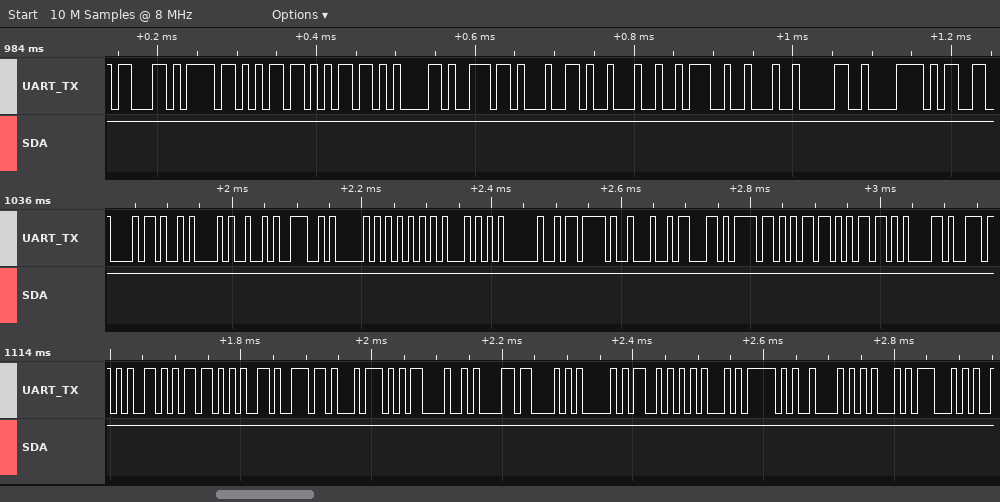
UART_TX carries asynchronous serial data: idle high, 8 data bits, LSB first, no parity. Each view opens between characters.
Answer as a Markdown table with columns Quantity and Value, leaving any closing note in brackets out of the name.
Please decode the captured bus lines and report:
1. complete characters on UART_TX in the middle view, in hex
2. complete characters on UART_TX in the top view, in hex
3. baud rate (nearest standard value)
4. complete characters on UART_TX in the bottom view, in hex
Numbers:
| Quantity | Value |
|---|---|
| complete characters on UART_TX in the middle view, in hex | 68, 0A, 49, 4E, 50, 55, 54, 20, 7B, 22, 63, 6F, 6D, 6D, 61 |
| complete characters on UART_TX in the top view, in hex | 63, 6F, 6D, 6D, 61, 6E, 64, 22, 3A, 22, 30, 78 |
| baud rate | 115200 baud |
| complete characters on UART_TX in the bottom view, in hex | 65, 6D, 65, 6E, 74, 0D, 0A, 43, 41, 53, 45, 5F, 42, 45, 47 |
